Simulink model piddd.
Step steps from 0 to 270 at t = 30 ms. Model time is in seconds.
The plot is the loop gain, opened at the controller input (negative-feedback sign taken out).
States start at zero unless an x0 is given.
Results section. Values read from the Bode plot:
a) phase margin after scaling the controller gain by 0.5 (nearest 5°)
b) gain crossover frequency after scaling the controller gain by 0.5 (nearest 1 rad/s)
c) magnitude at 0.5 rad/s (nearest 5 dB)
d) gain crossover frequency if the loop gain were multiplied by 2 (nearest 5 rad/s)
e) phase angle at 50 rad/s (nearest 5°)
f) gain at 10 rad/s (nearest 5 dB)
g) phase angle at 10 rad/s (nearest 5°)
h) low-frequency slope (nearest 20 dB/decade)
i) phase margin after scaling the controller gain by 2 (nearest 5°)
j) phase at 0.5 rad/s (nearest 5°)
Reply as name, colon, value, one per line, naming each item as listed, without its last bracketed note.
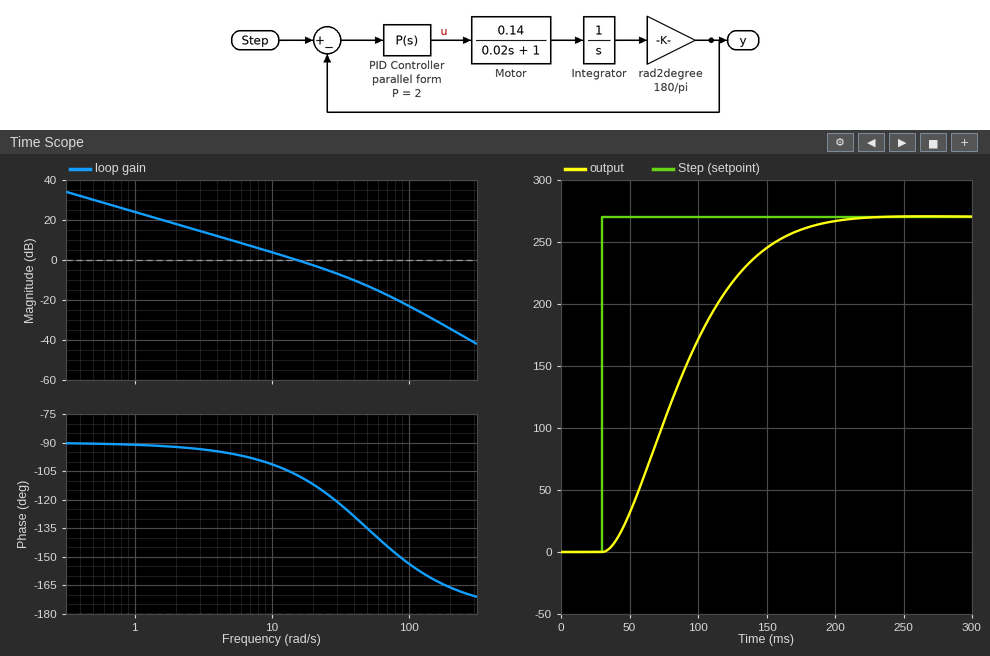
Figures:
phase margin after scaling the controller gain by 0.5: 80°
gain crossover frequency after scaling the controller gain by 0.5: 8 rad/s
magnitude at 0.5 rad/s: 30 dB
gain crossover frequency if the loop gain were multiplied by 2: 30 rad/s
phase angle at 50 rad/s: -135°
gain at 10 rad/s: 5 dB
phase angle at 10 rad/s: -100°
low-frequency slope: -20 dB/decade
phase margin after scaling the controller gain by 2: 60°
phase at 0.5 rad/s: -90°
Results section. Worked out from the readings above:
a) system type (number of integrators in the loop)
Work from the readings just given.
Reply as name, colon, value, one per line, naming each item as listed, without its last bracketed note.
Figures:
system type: 1
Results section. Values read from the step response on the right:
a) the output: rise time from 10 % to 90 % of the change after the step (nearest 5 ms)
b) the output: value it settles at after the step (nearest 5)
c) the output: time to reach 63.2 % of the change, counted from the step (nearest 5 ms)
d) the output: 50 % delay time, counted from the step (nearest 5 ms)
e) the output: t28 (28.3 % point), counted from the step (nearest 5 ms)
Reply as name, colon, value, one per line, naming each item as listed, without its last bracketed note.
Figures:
the output: rise time from 10 % to 90 % of the change after the step: 100 ms
the output: value it settles at after the step: 270
the output: time to reach 63.2 % of the change, counted from the step: 70 ms
the output: 50 % delay time, counted from the step: 55 ms
the output: t28 (28.3 % point), counted from the step: 35 ms
